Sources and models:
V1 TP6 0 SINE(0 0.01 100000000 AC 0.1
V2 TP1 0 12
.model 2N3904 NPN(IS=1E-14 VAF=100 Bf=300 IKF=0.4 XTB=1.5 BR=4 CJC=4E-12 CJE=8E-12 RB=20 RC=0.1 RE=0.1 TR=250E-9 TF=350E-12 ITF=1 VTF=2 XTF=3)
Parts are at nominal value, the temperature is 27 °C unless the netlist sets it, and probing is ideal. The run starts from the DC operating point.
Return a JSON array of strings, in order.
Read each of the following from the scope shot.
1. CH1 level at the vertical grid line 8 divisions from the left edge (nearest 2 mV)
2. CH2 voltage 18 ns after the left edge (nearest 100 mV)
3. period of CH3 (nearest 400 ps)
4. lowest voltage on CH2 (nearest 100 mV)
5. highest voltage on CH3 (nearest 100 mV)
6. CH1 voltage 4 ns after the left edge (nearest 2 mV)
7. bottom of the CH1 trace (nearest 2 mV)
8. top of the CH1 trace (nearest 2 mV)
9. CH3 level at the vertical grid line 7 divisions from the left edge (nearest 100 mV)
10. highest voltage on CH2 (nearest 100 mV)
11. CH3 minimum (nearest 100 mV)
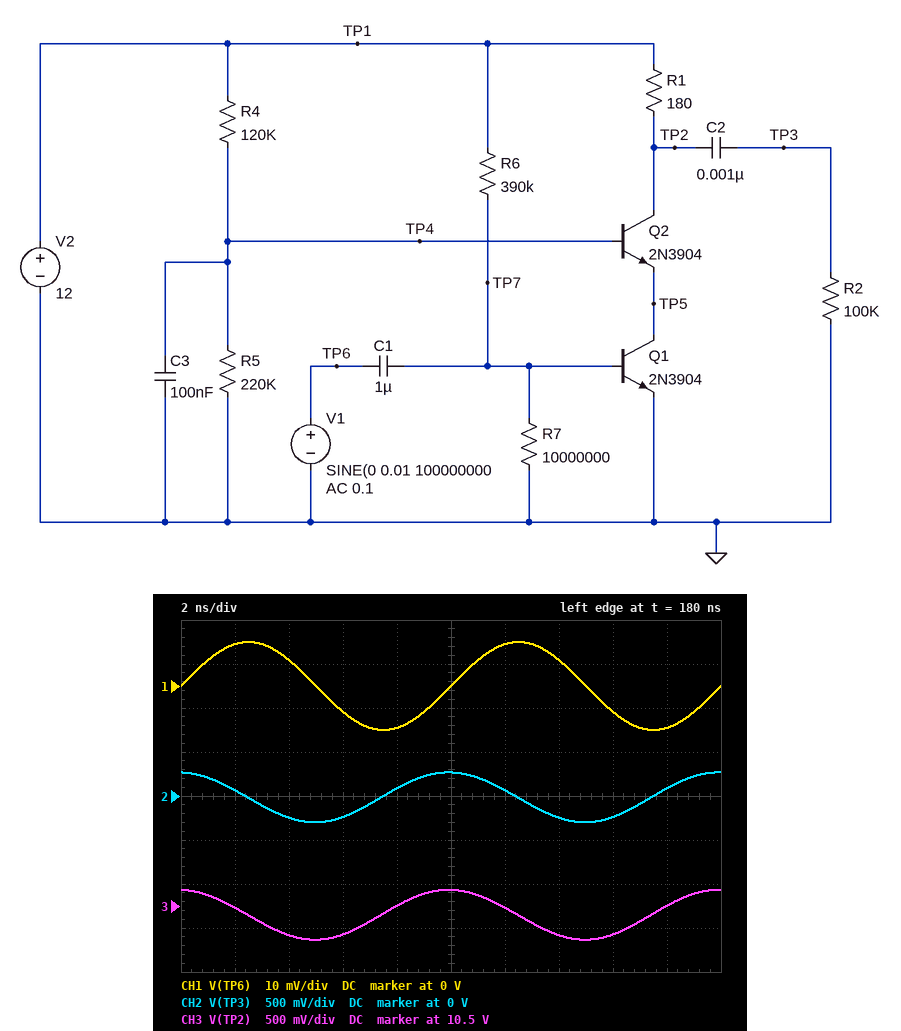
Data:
["-6 mV", "100 mV", "10.0 ns", "-300 mV", "10.7 V", "6 mV", "-10 mV", "10 mV", "10.2 V", "300 mV", "10.1 V"]
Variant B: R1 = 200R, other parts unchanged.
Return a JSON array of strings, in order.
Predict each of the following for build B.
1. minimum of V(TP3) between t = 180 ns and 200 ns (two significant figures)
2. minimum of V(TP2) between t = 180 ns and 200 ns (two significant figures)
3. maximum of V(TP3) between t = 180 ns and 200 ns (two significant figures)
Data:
["-330 mV", "9.9 V", "300 mV"]
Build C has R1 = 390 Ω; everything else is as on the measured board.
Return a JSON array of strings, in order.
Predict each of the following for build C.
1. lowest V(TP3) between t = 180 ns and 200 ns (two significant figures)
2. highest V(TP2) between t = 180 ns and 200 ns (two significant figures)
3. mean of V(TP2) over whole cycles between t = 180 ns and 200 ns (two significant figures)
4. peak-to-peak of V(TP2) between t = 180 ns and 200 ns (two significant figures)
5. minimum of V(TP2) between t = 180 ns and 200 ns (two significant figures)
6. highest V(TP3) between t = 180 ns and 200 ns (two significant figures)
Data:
["-560 mV", "9.1 V", "8.5 V", "1.1 V", "8.0 V", "510 mV"]
